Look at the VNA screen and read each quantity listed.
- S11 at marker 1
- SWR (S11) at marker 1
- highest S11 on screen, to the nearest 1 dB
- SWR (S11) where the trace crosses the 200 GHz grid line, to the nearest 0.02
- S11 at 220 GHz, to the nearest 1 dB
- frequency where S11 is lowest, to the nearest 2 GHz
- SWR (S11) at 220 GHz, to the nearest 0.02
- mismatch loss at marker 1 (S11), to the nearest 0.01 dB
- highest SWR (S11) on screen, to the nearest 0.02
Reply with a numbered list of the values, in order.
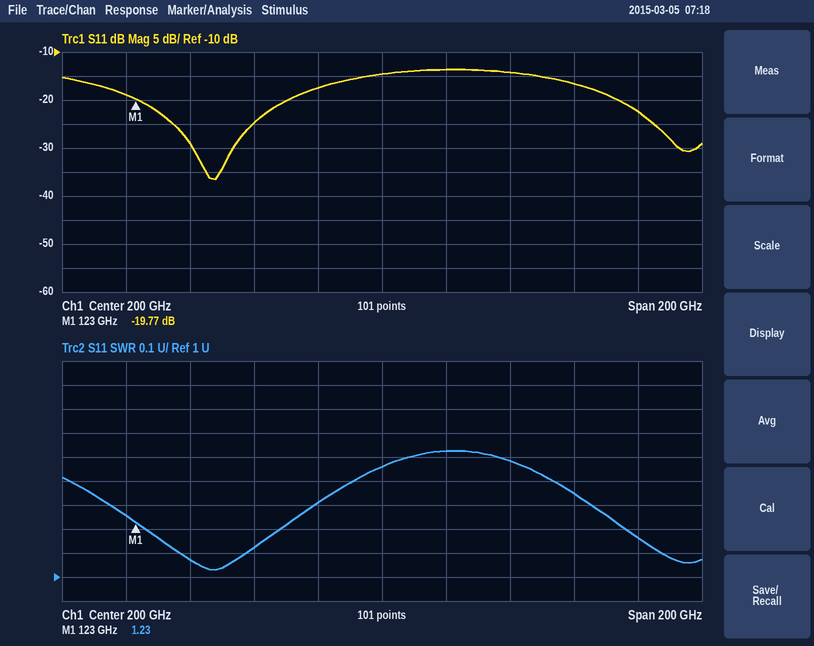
1. -19.77 dB
2. 1.23
3. -14 dB
4. 1.46
5. -14 dB
6. 148 GHz
7. 1.52
8. 0.05 dB
9. 1.52
